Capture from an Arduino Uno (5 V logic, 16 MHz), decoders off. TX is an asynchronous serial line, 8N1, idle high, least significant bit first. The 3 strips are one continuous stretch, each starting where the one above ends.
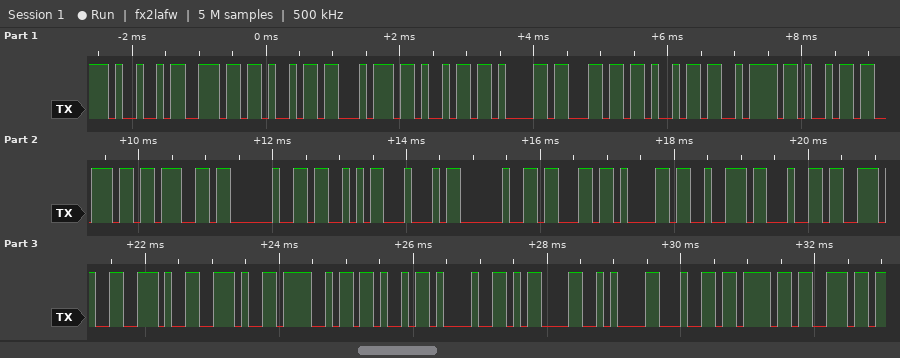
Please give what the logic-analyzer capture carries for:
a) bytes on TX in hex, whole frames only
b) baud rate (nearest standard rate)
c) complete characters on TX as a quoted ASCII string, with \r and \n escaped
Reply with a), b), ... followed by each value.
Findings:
a) 49 6E 69 74 69 61 6C 69 7A 69 6E 67 20 53 44 20 63 61 72 64 2E 2E 2E 4F 4B 21 0D 0A 64 6F 6E
b) 9600 baud
c) "Initializing SD card...OK!\r\ndon"
